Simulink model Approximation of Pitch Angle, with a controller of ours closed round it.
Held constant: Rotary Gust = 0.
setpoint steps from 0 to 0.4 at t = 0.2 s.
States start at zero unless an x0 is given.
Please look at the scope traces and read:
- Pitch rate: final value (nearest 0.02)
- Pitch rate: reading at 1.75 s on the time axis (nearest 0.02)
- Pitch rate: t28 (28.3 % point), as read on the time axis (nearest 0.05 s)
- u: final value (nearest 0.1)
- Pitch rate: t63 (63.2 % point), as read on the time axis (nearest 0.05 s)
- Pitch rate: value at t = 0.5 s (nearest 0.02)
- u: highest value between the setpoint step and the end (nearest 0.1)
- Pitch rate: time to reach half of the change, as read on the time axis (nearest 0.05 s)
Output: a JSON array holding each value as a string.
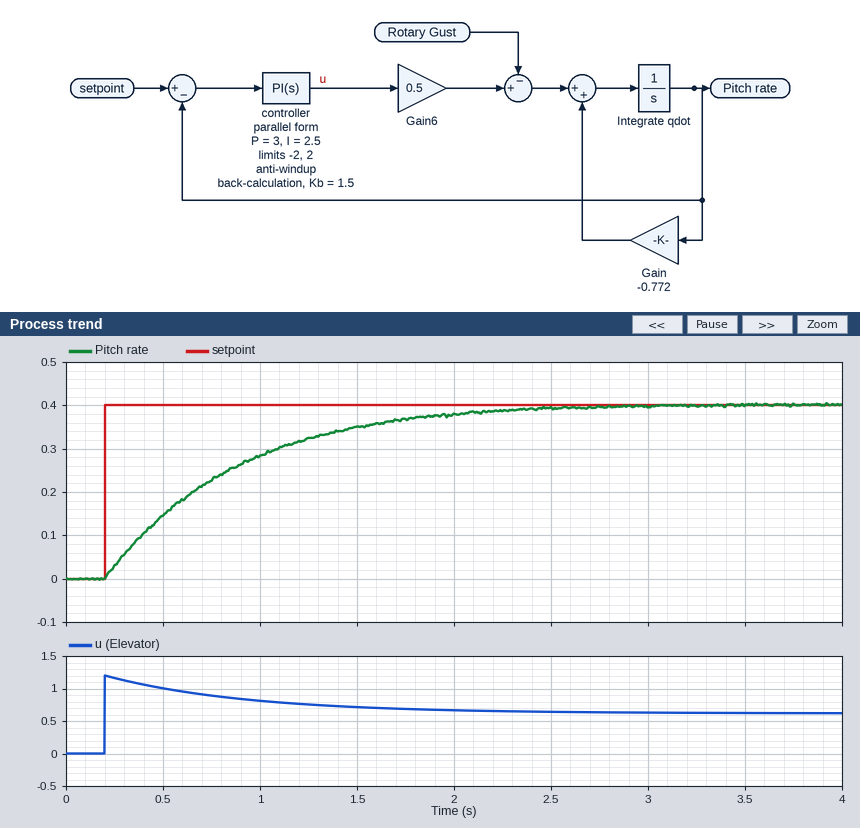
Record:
["0.40", "0.36", "0.40 s", "0.6", "0.85 s", "0.14", "1.2", "0.65 s"]
